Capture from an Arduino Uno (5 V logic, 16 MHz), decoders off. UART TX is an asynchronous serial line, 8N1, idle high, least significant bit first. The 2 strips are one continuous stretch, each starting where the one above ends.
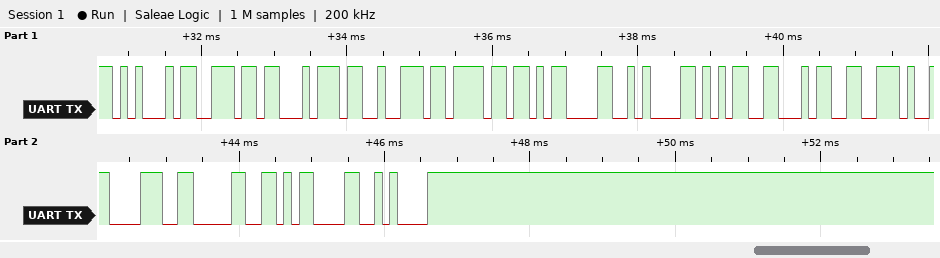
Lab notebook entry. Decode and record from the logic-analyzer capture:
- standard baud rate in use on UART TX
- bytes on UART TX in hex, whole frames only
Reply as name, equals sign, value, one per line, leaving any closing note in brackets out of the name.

standard baud rate in use on UART TX = 9600 baud
bytes on UART TX in hex, whole frames only = 0x45 0x6E 0x74 0x72 0x6F 0x0D 0x0A 0x35 0x34 0x2E 0x38 0x30 0x0D 0x0A
